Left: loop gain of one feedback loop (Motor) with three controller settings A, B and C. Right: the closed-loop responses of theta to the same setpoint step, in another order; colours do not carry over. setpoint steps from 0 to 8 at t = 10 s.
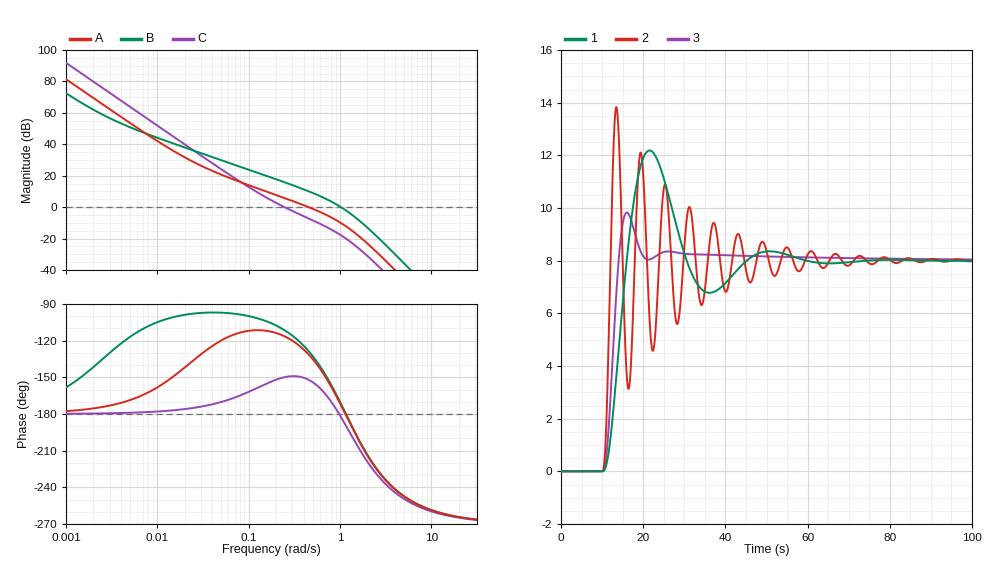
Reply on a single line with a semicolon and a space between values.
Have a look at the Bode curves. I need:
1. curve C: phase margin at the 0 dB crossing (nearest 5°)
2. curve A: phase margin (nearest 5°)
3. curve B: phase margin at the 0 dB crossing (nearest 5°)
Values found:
30°; 50°; 10°
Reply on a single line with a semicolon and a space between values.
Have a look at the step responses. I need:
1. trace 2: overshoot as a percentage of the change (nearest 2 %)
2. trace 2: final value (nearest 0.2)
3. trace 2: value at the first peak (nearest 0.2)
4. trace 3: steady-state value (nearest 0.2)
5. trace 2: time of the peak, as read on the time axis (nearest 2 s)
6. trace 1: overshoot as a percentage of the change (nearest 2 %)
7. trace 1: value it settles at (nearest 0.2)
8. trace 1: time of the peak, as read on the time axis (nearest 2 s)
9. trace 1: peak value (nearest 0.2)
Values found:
72 %; 8.0; 13.8; 8.0; 14 s; 52 %; 8.0; 22 s; 12.2
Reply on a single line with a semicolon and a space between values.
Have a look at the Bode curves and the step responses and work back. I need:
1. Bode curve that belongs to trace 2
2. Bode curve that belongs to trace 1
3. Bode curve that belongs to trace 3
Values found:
B; C; A
